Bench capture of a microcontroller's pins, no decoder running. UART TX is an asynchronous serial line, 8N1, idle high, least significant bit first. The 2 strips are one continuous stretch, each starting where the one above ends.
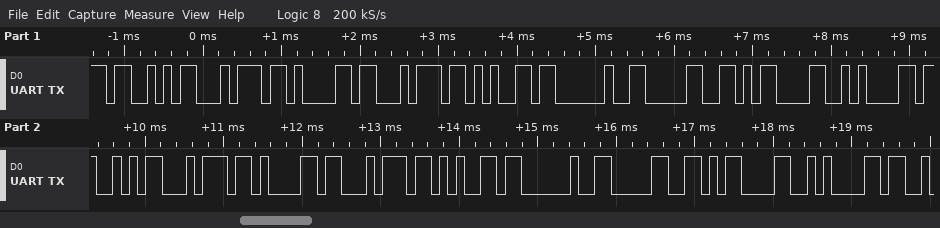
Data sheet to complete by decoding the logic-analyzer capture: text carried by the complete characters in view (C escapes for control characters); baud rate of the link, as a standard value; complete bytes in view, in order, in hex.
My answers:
"State 0\r\nState 0\r\n"
9600 baud
53 74 61 74 65 20 30 0D 0A 53 74 61 74 65 20 30 0D 0A
